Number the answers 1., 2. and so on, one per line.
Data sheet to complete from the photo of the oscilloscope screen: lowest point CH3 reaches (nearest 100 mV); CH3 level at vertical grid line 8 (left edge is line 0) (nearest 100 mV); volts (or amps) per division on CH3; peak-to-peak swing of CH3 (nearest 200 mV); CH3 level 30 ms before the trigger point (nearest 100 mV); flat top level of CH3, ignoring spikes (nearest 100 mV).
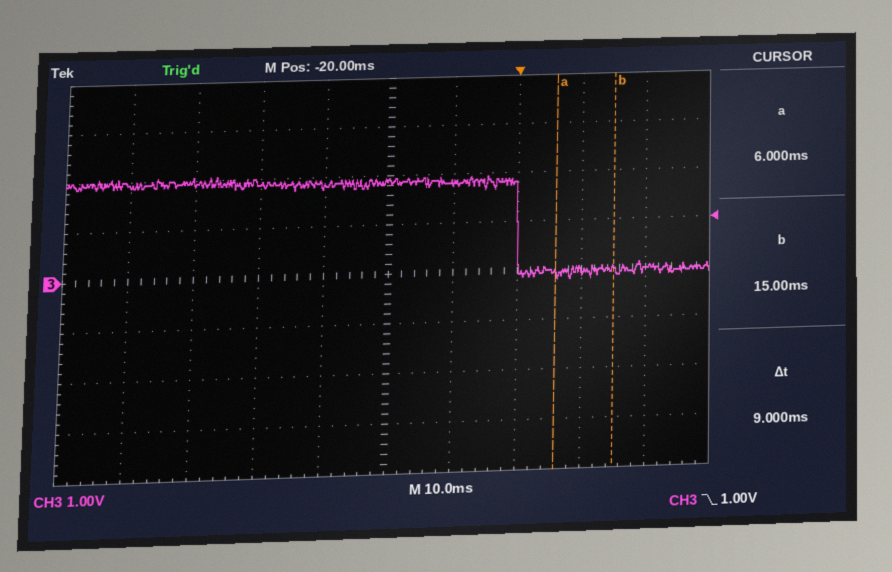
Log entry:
1. -200 mV
2. 0.0 V
3. 1 V
4. 2.2 V
5. 1.8 V
6. 1.9 V
